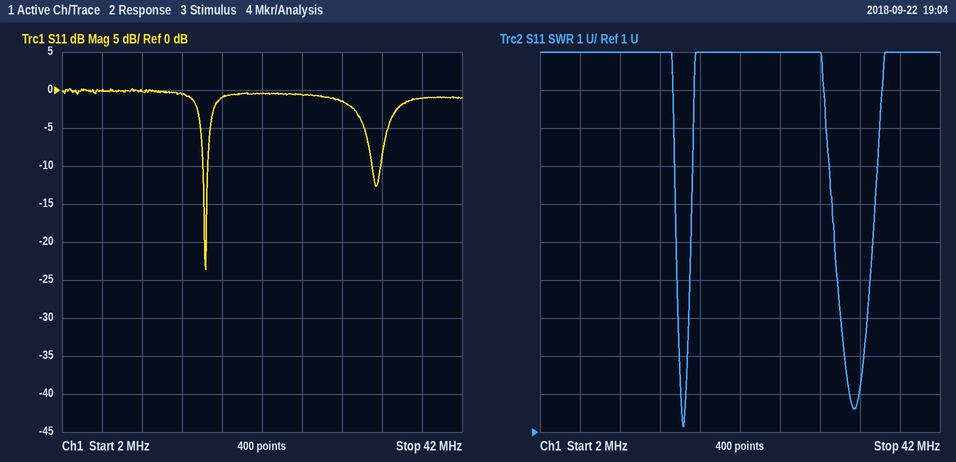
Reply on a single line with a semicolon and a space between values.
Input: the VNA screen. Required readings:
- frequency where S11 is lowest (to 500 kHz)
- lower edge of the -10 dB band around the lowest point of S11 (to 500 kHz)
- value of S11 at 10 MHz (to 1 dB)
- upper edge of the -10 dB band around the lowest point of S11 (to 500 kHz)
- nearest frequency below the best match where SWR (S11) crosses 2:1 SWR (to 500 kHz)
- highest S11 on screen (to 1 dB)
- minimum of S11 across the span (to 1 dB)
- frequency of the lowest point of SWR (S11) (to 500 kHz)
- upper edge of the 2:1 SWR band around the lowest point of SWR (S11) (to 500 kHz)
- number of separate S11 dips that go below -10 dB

16.5 MHz; 16.0 MHz; 0 dB; 16.5 MHz; 16.0 MHz; 0 dB; -24 dB; 16.5 MHz; 16.5 MHz; 2
